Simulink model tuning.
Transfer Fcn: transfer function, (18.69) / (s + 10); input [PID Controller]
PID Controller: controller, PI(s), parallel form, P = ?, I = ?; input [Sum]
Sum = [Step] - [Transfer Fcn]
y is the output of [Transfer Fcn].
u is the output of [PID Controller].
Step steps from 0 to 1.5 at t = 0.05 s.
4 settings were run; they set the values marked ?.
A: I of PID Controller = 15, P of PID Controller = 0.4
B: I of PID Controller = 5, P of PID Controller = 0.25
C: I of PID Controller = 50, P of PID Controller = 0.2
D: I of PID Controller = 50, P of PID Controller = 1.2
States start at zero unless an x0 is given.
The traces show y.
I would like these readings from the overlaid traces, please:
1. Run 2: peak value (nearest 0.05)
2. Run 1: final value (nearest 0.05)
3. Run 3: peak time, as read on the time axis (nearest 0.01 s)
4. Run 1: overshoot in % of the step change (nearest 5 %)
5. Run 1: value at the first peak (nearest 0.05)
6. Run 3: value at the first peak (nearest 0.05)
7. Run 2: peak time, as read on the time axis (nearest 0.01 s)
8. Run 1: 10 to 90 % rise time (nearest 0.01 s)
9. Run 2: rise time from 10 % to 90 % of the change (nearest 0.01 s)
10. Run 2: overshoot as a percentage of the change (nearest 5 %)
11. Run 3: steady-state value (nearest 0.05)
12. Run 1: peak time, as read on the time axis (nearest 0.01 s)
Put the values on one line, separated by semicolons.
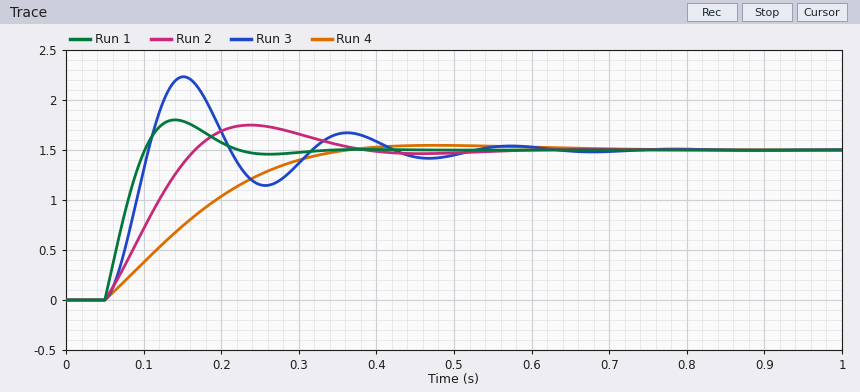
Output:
1.75; 1.50; 0.15 s; 20 %; 1.80; 2.25; 0.24 s; 0.04 s; 0.09 s; 15 %; 1.50; 0.14 s
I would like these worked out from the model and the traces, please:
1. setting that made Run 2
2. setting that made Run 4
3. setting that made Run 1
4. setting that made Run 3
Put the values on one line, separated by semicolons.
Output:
A; B; D; C
